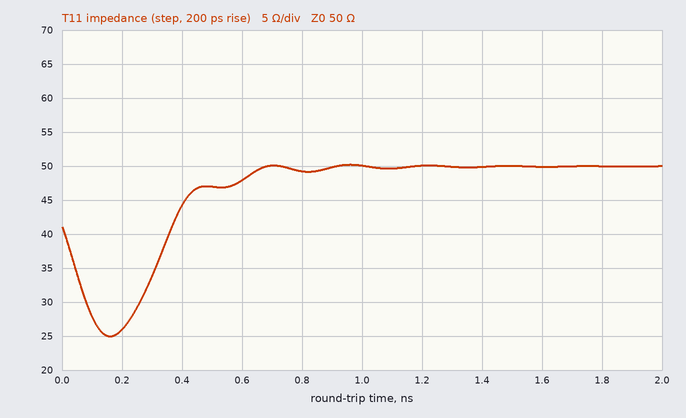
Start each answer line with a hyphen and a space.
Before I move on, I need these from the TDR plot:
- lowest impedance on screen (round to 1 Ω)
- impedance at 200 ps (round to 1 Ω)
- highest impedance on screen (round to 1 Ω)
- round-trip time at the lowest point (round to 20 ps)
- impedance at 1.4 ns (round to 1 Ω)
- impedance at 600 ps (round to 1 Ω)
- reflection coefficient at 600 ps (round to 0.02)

- 25 Ω
- 26 Ω
- 50 Ω
- 160 ps
- 50 Ω
- 48 Ω
- -0.02
